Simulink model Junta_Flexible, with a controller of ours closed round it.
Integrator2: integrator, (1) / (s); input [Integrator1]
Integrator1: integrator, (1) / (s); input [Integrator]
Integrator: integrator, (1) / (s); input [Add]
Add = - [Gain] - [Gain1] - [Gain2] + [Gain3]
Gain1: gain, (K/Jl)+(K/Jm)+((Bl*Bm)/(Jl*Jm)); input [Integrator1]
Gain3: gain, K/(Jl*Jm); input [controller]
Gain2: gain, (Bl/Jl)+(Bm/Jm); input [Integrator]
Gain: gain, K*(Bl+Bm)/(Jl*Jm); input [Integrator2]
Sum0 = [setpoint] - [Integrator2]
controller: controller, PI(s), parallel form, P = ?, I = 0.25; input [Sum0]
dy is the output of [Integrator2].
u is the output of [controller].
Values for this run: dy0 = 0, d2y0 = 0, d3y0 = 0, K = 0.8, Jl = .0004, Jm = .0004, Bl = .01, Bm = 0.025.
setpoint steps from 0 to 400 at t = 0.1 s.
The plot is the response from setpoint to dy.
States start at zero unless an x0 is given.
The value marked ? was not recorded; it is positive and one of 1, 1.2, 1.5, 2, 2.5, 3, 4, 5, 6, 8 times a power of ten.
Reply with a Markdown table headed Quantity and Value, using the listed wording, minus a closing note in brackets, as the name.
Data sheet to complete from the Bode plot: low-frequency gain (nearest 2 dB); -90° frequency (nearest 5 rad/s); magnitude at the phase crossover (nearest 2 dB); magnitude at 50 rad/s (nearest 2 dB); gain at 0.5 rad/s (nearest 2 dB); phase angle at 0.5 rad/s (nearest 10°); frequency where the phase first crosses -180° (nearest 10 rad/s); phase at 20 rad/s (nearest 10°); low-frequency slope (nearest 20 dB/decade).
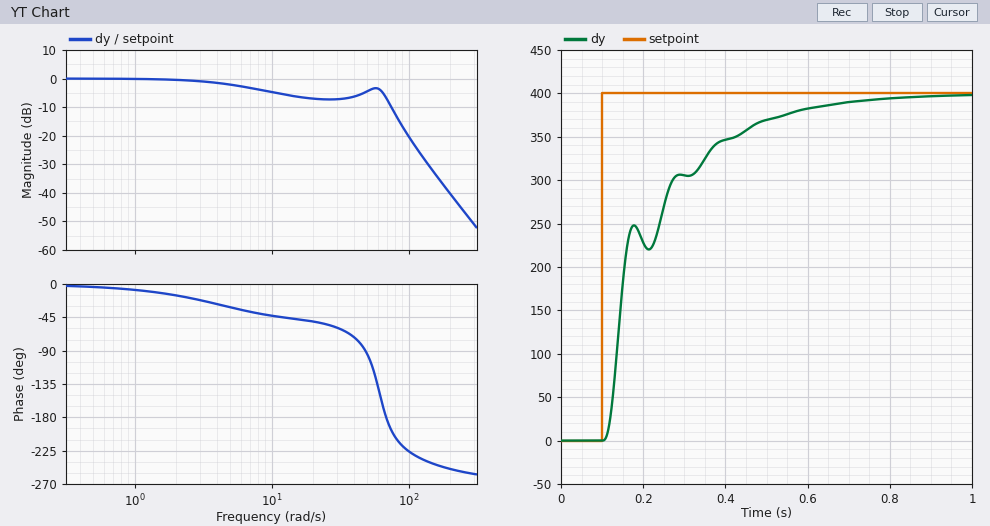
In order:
| Quantity | Value |
|---|---|
| low-frequency gain | 0 dB |
| -90° frequency | 50 rad/s |
| magnitude at the phase crossover | -6 dB |
| magnitude at 50 rad/s | -4 dB |
| gain at 0.5 rad/s | 0 dB |
| phase angle at 0.5 rad/s | 0° |
| frequency where the phase first crosses -180° | 70 rad/s |
| phase at 20 rad/s | -50° |
| low-frequency slope | 0 dB/decade |
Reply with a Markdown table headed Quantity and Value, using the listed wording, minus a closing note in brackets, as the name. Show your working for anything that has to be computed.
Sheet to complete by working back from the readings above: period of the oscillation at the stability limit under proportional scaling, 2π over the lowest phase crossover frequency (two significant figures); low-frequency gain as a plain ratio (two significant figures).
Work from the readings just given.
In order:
| Quantity | Value |
|---|---|
| period of the oscillation at the stability limit under proportional scaling, 2π over the lowest phase crossover frequency | 2π / 70 = 0.090 s |
| low-frequency gain as a plain ratio | 10^(0 / 20) = 1.0 |
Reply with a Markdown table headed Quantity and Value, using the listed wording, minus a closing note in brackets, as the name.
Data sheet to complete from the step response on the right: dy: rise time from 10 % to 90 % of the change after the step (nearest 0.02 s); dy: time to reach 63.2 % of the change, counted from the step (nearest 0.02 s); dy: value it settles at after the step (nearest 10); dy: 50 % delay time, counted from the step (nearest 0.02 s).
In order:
| Quantity | Value |
|---|---|
| dy: rise time from 10 % to 90 % of the change after the step | 0.34 s |
| dy: time to reach 63.2 % of the change, counted from the step | 0.14 s |
| dy: value it settles at after the step | 400 |
| dy: 50 % delay time, counted from the step | 0.06 s |
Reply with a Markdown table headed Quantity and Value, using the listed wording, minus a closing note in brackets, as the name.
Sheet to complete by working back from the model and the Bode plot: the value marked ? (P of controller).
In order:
| Quantity | Value |
|---|---|
| the value marked ? | 0.015 |
